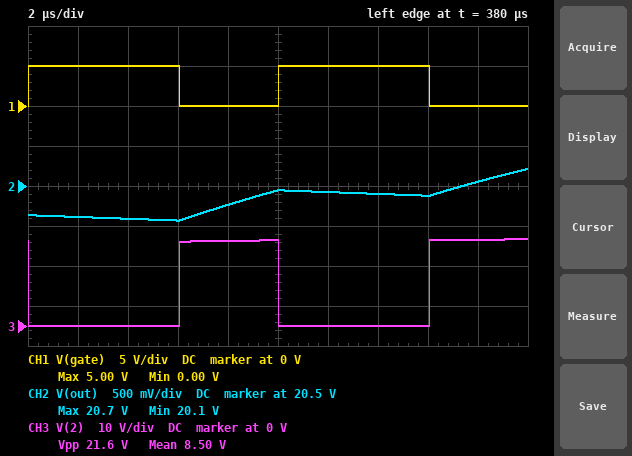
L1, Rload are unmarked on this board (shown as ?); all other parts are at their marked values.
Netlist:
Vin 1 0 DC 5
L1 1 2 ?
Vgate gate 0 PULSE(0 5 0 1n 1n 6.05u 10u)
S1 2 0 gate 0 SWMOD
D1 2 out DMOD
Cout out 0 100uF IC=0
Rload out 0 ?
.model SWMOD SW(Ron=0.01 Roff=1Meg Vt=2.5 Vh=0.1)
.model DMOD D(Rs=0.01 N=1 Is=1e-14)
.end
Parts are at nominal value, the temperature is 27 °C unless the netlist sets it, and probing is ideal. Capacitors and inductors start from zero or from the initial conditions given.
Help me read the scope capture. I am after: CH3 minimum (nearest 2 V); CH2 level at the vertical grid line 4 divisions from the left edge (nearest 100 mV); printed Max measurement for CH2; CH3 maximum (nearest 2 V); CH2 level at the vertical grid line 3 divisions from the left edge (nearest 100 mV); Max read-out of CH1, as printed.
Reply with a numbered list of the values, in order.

1. 0 V
2. 20.3 V
3. 20.7 V
4. 22 V
5. 20.1 V
6. 5.00 V
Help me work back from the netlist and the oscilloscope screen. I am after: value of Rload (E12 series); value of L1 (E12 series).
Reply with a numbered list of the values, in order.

1. 18 Ω
2. 33 µH
